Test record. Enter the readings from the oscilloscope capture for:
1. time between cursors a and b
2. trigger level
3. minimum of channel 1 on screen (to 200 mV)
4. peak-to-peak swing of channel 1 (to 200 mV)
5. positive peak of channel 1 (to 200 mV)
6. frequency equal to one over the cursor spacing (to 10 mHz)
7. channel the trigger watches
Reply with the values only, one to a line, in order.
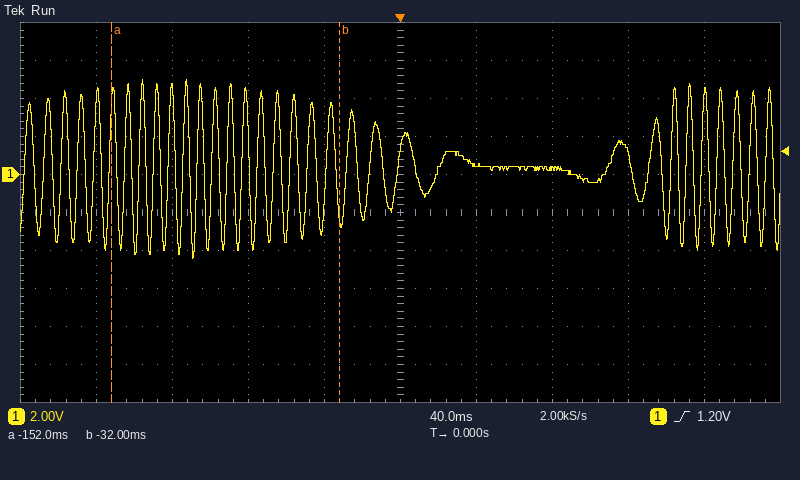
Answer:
120 ms
1.20 V
-4.4 V
9.4 V
5.0 V
8.33 Hz
channel 1
